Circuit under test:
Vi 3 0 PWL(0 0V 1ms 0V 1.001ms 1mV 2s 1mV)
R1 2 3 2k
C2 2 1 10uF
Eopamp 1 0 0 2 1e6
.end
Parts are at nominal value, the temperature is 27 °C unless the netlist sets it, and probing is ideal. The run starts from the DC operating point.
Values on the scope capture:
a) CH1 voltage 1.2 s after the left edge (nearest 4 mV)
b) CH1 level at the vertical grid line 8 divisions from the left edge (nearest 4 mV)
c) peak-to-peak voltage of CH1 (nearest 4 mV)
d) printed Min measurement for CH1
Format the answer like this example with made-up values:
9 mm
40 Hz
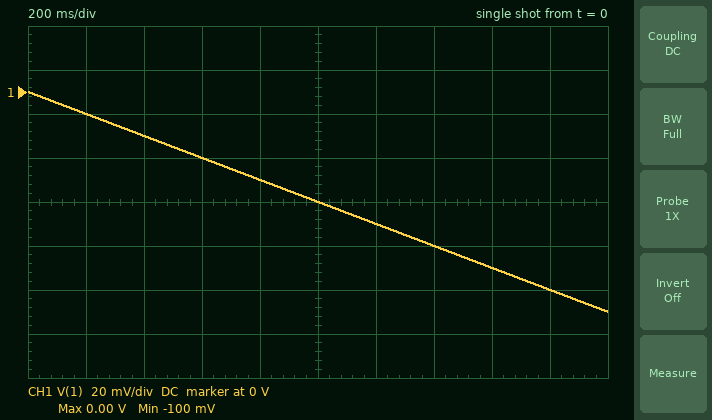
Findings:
-60 mV
-80 mV
100 mV
-100 mV
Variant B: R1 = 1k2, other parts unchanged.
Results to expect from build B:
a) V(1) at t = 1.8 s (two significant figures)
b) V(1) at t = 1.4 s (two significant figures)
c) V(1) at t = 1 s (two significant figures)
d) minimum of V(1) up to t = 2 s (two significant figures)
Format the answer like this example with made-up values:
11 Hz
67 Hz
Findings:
-150 mV
-120 mV
-83 mV
-170 mV
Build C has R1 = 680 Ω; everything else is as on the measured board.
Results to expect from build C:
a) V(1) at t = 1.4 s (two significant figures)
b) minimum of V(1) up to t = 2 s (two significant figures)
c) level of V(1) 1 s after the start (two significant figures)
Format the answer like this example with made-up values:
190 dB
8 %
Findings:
-210 mV
-290 mV
-150 mV
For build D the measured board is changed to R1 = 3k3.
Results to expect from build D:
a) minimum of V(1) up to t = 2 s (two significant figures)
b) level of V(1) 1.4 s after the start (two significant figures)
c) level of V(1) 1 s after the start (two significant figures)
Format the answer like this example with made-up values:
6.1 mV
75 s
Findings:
-61 mV
-42 mV
-30 mV
